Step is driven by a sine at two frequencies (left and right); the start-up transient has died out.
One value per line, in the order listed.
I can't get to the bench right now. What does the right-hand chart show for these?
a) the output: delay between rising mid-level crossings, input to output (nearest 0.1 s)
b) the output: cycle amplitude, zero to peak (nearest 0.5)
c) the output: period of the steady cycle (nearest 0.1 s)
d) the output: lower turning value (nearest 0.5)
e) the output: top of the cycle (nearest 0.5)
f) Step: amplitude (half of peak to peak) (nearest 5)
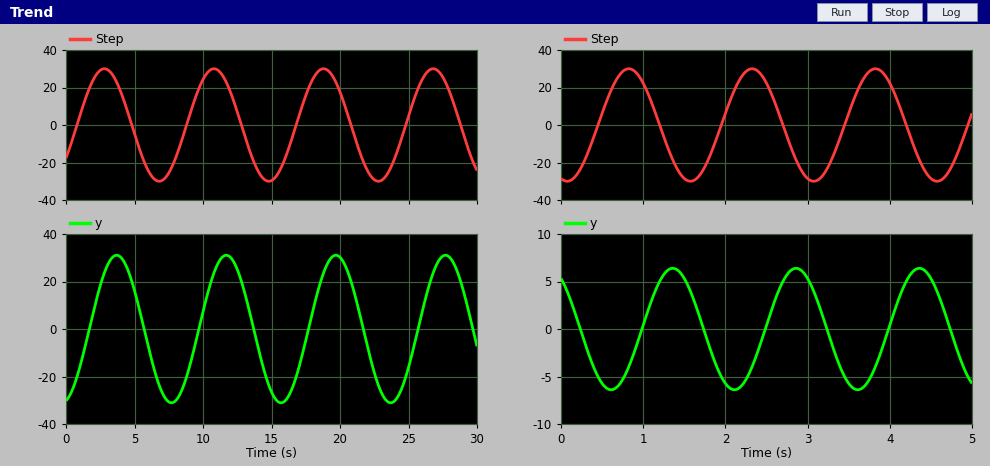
0.5 s
6.5
1.5 s
-6.5
6.5
30
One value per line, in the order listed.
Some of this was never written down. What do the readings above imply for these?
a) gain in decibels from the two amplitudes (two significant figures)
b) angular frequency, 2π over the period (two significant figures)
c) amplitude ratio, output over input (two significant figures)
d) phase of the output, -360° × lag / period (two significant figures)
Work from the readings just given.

-13 dB
4.2 rad/s
0.22
-120°
